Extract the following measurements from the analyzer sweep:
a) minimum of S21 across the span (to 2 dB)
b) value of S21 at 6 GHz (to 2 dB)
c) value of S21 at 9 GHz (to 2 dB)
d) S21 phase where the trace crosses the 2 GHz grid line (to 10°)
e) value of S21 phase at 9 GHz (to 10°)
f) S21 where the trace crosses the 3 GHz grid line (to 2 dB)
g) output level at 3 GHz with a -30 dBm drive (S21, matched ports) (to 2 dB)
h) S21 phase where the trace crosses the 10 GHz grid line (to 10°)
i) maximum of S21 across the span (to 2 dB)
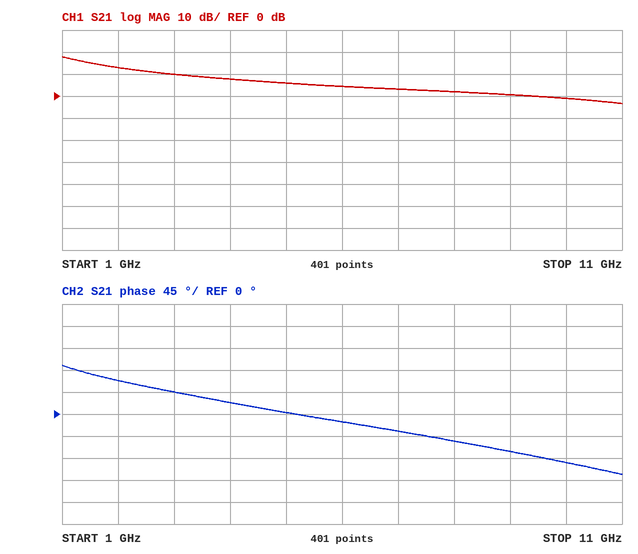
-4 dB
4 dB
0 dB
70°
-80°
10 dB
-20 dBm
-100°
18 dB
